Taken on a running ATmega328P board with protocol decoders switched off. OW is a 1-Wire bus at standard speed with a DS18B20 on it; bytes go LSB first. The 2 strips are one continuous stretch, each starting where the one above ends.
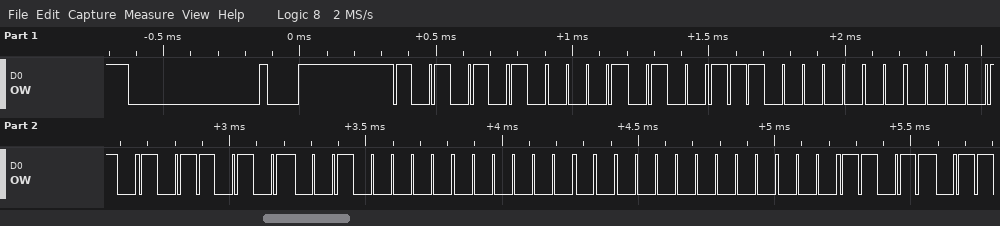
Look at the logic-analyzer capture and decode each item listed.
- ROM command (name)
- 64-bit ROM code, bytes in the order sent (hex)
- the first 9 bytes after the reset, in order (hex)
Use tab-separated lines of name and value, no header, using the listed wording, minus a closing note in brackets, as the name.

ROM command	Match ROM
64-bit ROM code, bytes in the order sent	28 07 40 AD 04 00 00 D8
the first 9 bytes after the reset, in order	55 28 07 40 AD 04 00 00 D8
